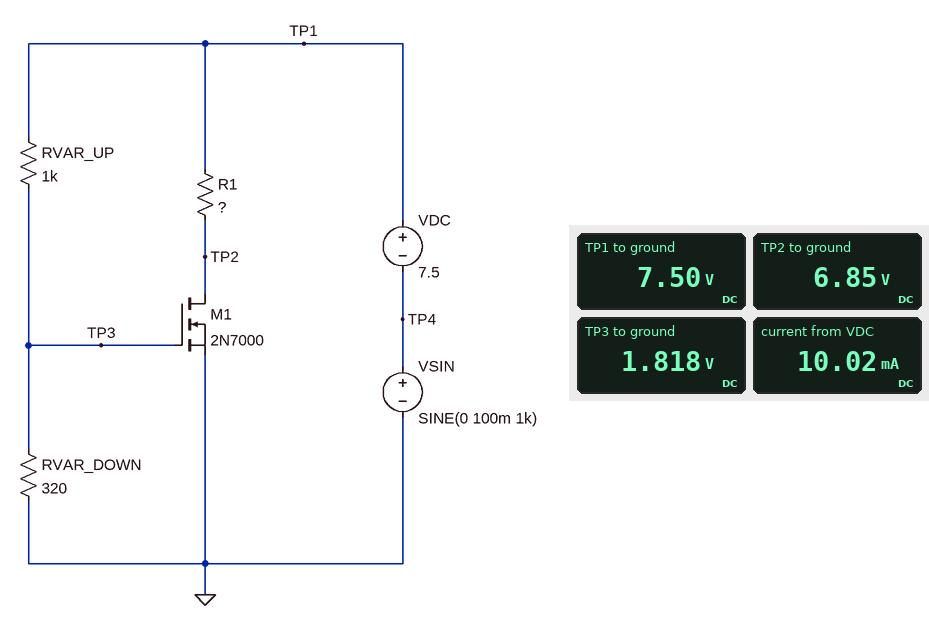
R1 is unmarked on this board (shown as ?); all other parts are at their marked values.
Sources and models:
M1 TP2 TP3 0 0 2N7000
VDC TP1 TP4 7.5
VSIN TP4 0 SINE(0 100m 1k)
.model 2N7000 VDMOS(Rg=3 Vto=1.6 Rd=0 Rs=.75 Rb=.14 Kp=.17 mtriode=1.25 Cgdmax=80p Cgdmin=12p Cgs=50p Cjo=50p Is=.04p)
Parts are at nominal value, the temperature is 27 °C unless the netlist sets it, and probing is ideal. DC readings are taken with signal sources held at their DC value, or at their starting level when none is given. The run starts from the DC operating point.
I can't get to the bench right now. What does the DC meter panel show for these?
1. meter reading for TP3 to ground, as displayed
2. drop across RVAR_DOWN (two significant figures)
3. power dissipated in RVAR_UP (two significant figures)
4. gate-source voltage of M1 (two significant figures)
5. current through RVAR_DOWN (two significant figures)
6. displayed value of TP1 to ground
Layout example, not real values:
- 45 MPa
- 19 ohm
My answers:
- 1.818 V
- 1.8 V
- 32 mW
- 1.8 V
- 5.7 mA
- 7.50 V
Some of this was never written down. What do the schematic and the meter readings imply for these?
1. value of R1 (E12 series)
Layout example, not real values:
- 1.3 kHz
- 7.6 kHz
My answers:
- 150 Ω
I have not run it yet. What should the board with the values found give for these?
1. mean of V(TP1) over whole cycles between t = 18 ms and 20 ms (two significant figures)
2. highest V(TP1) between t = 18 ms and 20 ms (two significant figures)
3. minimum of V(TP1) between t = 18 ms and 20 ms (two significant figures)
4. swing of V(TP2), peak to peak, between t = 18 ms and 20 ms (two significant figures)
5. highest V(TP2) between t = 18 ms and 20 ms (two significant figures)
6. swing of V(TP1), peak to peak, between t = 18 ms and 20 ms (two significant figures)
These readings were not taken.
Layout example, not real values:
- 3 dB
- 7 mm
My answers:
- 7.5 V
- 7.6 V
- 7.4 V
- 44 mV
- 6.9 V
- 200 mV
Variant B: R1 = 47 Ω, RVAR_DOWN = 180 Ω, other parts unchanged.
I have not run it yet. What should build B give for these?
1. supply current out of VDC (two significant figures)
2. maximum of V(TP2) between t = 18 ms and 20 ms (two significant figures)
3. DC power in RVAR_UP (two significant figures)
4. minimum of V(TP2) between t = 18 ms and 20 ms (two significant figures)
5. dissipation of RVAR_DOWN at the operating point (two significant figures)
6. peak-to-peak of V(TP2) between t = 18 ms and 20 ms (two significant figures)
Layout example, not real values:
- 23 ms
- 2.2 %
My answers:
- 6.4 mA
- 7.6 V
- 40 mW
- 7.4 V
- 7.3 mW
- 200 mV
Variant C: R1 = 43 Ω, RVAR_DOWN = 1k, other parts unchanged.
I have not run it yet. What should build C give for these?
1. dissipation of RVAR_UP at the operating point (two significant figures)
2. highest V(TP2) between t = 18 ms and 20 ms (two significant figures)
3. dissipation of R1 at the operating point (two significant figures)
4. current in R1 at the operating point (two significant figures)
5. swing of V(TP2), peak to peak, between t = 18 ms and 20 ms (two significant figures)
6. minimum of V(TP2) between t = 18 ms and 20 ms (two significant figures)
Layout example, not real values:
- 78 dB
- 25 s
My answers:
- 14 mW
- 560 mV
- 1.1 W
- 160 mA
- 9.0 mV
- 550 mV
